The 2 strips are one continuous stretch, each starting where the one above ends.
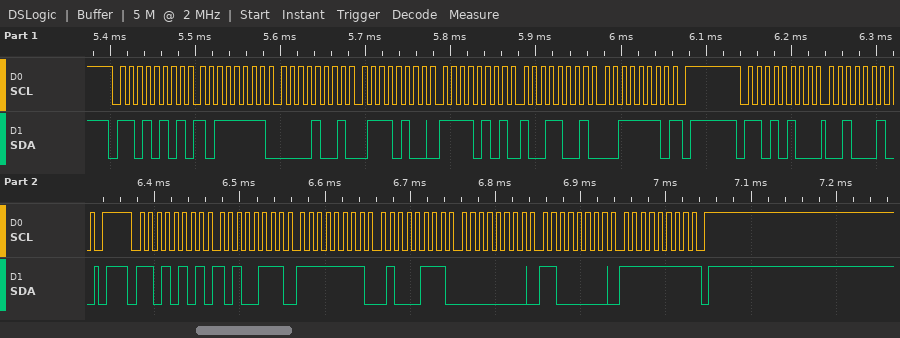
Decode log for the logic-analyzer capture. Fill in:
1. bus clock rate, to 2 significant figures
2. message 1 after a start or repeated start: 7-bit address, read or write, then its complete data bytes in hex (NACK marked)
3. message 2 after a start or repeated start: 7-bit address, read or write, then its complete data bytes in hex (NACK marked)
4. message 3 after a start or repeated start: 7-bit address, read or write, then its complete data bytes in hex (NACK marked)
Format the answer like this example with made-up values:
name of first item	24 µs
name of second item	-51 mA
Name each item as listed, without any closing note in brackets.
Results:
bus clock rate, to 2 significant figures	100 kHz
message 1 after a start or repeated start: 7-bit address, read or write, then its complete data bytes in hex	0x6A read: BF 09 74 F5 99 3E NACK
message 2 after a start or repeated start: 7-bit address, read or write, then its complete data bytes in hex	0x6A write: 22
message 3 after a start or repeated start: 7-bit address, read or write, then its complete data bytes in hex	0x6A read: A7 FF 47 00 C0 FF NACK
